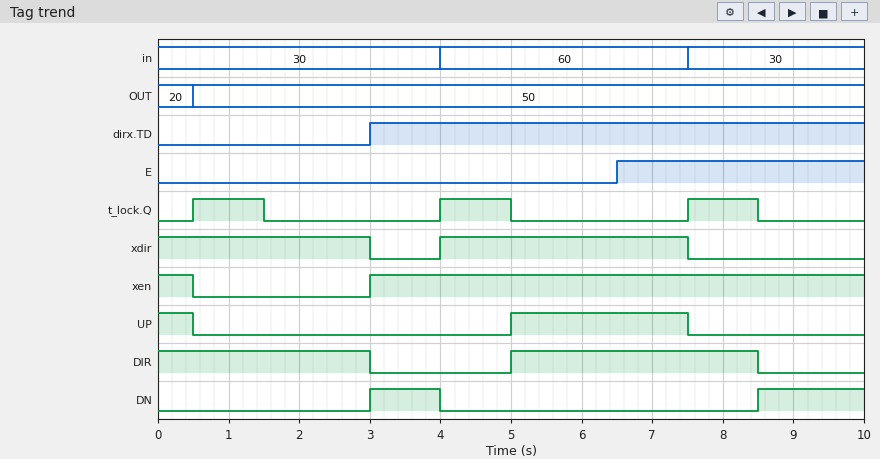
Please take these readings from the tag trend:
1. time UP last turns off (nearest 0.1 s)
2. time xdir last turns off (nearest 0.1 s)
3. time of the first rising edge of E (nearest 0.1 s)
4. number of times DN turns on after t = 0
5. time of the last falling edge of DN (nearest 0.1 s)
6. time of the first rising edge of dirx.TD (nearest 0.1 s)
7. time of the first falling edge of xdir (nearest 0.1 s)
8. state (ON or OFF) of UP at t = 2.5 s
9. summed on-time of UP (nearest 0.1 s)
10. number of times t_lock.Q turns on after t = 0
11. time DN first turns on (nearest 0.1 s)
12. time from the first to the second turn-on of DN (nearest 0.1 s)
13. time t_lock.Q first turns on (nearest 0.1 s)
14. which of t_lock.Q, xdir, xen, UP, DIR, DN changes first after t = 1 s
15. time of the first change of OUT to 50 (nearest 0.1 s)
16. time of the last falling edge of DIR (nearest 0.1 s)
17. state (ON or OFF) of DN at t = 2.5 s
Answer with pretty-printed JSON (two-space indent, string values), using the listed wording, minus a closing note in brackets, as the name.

{
  "time UP last turns off": "7.5 s",
  "time xdir last turns off": "7.5 s",
  "time of the first rising edge of E": "6.5 s",
  "number of times DN turns on after t = 0": "2",
  "time of the last falling edge of DN": "4.0 s",
  "time of the first rising edge of dirx.TD": "3.0 s",
  "time of the first falling edge of xdir": "3.0 s",
  "state (ON or OFF) of UP at t = 2.5 s": "OFF",
  "summed on-time of UP": "3.0 s",
  "number of times t_lock.Q turns on after t = 0": "3",
  "time DN first turns on": "3.0 s",
  "time from the first to the second turn-on of DN": "5.5 s",
  "time t_lock.Q first turns on": "0.5 s",
  "which of t_lock.Q, xdir, xen, UP, DIR, DN changes first after t = 1 s": "t_lock.Q",
  "time of the first change of OUT to 50": "0.5 s",
  "time of the last falling edge of DIR": "8.5 s",
  "state (ON or OFF) of DN at t = 2.5 s": "OFF"
}
